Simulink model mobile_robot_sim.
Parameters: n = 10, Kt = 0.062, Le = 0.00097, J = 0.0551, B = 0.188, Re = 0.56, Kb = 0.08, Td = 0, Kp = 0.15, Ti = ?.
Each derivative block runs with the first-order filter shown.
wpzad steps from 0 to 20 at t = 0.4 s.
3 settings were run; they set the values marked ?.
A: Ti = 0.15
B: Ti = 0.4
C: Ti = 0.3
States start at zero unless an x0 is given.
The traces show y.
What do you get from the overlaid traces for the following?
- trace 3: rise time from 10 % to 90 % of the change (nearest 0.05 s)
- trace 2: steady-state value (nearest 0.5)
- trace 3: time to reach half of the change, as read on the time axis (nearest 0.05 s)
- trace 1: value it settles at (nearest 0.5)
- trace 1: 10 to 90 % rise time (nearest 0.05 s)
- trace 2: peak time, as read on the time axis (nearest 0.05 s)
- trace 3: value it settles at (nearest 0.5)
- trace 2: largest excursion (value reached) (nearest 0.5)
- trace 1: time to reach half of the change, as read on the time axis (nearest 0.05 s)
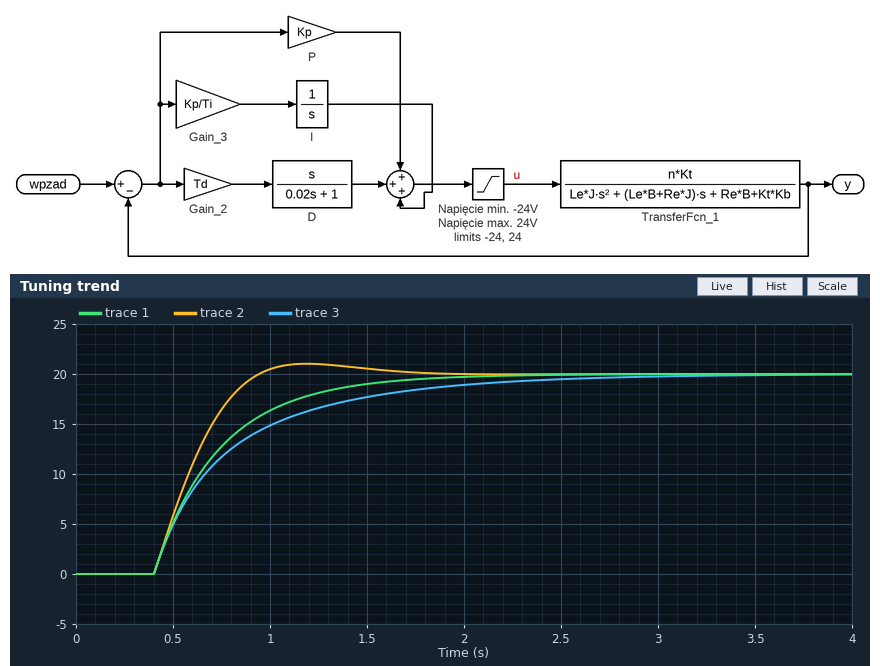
1.15 s
20.0
0.65 s
20.0
0.80 s
1.20 s
20.0
21.0
0.65 s
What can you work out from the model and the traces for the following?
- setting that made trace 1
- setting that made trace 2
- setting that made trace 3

C
A
B
